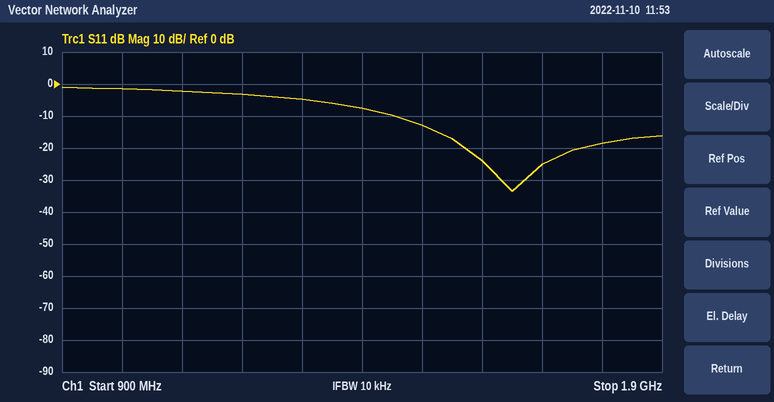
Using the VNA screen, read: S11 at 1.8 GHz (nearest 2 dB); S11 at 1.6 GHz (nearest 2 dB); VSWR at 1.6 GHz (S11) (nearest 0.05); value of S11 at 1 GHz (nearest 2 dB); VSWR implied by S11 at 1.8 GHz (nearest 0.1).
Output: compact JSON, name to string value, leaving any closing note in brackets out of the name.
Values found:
{"S11 at 1.8 GHz": "-18 dB", "S11 at 1.6 GHz": "-24 dB", "VSWR at 1.6 GHz (S11)": "1.15", "value of S11 at 1 GHz": "-2 dB", "VSWR implied by S11 at 1.8 GHz": "1.3"}
